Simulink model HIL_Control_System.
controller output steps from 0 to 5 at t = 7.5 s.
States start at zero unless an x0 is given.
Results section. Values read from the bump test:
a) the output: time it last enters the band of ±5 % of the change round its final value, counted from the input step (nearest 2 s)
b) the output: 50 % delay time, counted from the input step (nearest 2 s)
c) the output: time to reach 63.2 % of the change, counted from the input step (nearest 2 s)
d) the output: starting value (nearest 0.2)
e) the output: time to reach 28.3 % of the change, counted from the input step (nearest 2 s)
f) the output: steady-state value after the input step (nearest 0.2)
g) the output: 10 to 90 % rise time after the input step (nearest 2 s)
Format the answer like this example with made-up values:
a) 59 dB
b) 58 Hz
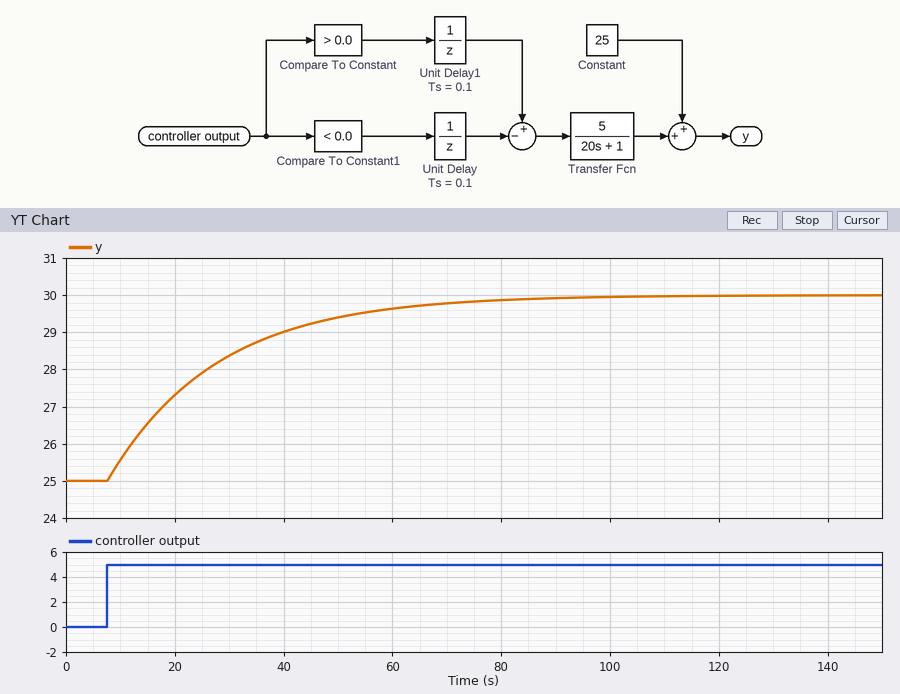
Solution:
a) 60 s
b) 14 s
c) 20 s
d) 25.0
e) 6 s
f) 30.0
g) 44 s
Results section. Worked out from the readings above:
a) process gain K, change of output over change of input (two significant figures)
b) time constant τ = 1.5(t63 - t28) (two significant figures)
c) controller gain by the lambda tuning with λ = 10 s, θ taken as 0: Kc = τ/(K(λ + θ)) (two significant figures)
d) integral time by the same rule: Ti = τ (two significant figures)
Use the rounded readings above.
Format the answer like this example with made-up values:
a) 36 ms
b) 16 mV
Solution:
a) 1.0
b) 21 s
c) 2.1
d) 21 s
